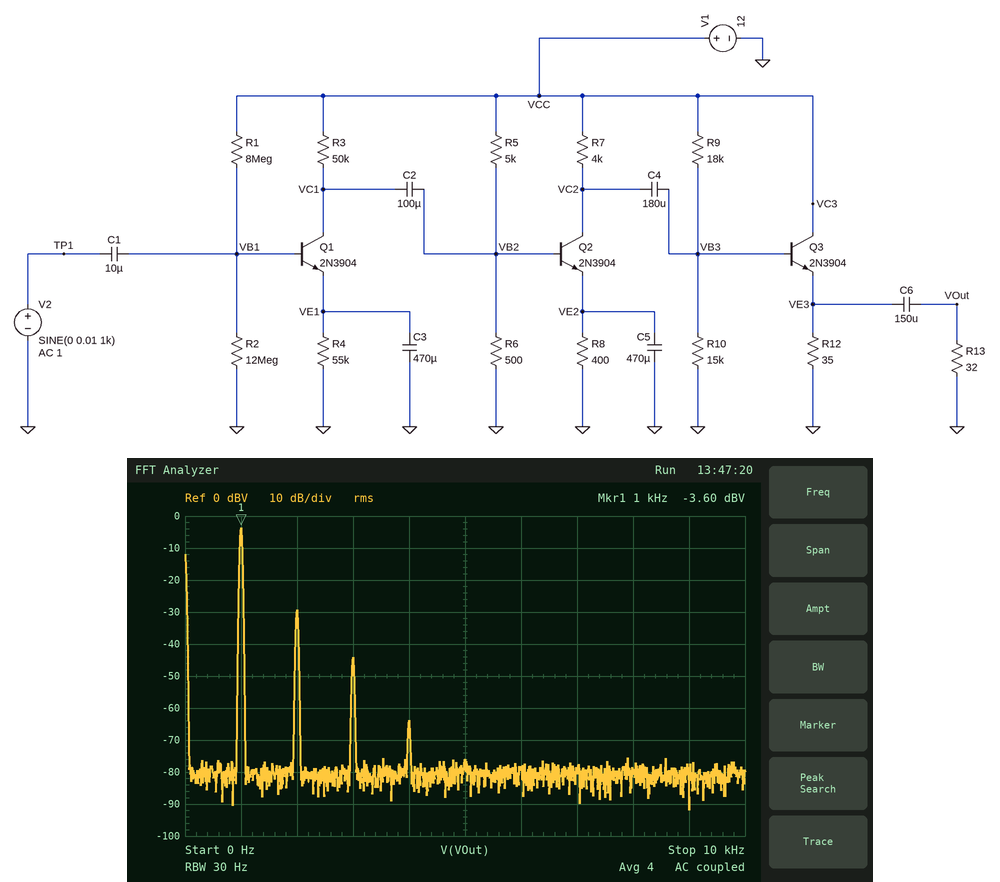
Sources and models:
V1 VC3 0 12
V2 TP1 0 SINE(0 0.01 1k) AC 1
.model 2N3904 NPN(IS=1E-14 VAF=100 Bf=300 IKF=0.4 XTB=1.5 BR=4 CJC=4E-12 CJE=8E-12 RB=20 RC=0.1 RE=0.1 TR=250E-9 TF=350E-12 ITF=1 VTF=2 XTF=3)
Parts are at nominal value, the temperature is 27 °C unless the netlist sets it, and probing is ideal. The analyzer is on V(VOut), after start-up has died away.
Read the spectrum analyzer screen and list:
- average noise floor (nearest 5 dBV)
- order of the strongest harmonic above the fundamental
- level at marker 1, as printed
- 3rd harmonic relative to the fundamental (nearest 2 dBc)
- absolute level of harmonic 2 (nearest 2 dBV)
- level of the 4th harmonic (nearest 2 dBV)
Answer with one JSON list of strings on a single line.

["-80 dBV", "2", "-3.60 dBV", "-40 dBc", "-30 dBV", "-64 dBV"]
